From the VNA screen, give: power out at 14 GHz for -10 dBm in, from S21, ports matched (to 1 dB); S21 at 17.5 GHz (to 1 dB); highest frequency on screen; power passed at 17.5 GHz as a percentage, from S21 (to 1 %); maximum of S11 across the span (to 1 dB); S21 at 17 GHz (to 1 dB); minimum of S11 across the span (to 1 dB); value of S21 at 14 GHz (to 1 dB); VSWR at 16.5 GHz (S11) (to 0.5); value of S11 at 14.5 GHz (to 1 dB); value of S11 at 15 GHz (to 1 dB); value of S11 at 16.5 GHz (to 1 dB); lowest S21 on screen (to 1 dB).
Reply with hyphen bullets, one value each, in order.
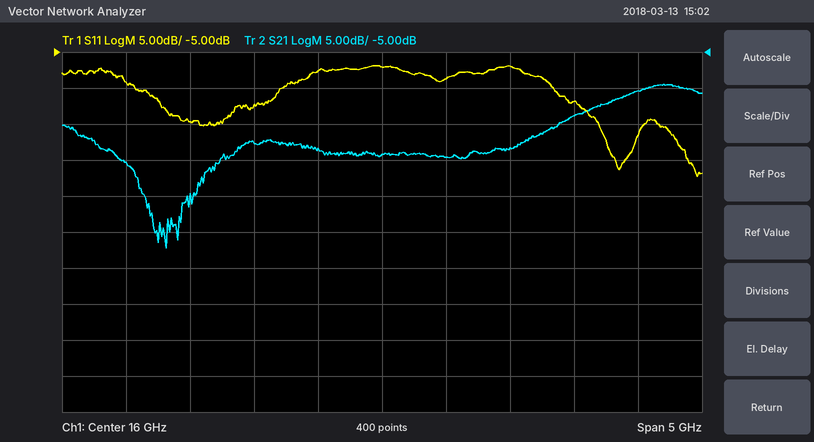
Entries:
- -30 dBm
- -14 dB
- 18.5 GHz
- 4 %
- -7 dB
- -18 dB
- -22 dB
- -20 dB
- 2.0
- -15 dB
- -12 dB
- -9 dB
- -32 dB
